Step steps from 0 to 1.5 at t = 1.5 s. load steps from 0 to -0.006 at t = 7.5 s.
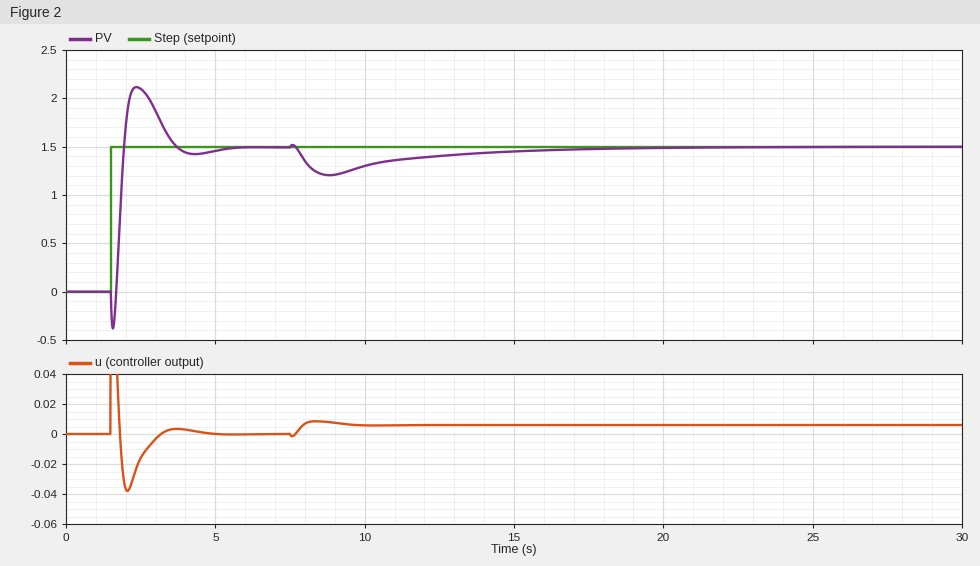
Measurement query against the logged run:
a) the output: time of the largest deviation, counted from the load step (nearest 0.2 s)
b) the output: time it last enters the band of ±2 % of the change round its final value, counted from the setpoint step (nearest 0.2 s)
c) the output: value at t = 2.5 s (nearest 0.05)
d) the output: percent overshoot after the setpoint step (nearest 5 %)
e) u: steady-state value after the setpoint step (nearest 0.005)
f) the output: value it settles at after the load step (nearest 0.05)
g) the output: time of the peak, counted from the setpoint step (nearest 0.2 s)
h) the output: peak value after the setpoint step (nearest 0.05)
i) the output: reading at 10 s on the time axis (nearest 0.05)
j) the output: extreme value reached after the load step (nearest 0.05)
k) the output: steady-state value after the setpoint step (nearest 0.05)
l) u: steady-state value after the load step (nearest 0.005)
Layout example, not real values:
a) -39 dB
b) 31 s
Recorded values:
a) 1.4 s
b) 3.8 s
c) 2.10
d) 40 %
e) 0.000
f) 1.50
g) 0.8 s
h) 2.10
i) 1.30
j) 1.20
k) 1.50
l) 0.005
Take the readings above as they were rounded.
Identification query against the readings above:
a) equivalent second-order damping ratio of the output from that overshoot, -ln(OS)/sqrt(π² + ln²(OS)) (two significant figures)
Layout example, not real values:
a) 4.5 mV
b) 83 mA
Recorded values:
a) 0.28
